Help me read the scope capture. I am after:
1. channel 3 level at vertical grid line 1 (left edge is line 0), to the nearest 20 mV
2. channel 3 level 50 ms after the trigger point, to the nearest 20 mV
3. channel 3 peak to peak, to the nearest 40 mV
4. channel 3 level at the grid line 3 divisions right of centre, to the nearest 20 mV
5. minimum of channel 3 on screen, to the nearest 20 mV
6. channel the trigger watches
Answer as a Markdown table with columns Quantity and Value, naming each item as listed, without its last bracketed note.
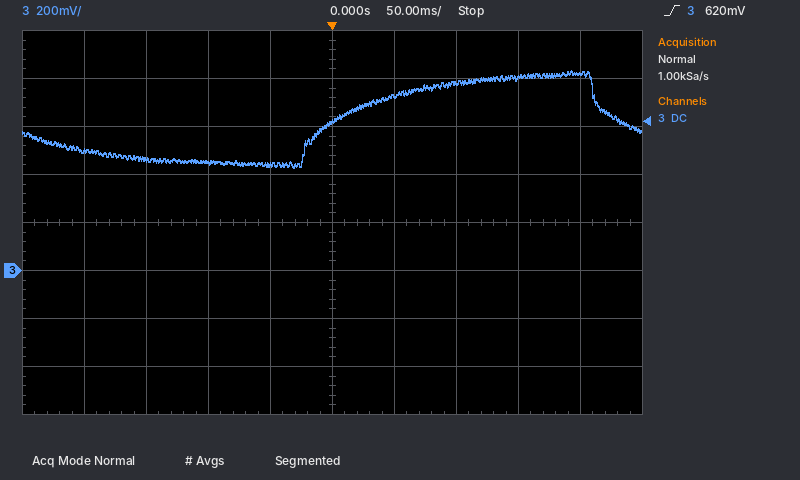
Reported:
| Quantity | Value |
|---|---|
| channel 3 level at vertical grid line 1 (left edge is line 0), to the nearest 20 mV | 500 mV |
| channel 3 level 50 ms after the trigger point, to the nearest 20 mV | 720 mV |
| channel 3 peak to peak, to the nearest 40 mV | 400 mV |
| channel 3 level at the grid line 3 divisions right of centre, to the nearest 20 mV | 800 mV |
| minimum of channel 3 on screen, to the nearest 20 mV | 420 mV |
| channel the trigger watches | channel 3 |
